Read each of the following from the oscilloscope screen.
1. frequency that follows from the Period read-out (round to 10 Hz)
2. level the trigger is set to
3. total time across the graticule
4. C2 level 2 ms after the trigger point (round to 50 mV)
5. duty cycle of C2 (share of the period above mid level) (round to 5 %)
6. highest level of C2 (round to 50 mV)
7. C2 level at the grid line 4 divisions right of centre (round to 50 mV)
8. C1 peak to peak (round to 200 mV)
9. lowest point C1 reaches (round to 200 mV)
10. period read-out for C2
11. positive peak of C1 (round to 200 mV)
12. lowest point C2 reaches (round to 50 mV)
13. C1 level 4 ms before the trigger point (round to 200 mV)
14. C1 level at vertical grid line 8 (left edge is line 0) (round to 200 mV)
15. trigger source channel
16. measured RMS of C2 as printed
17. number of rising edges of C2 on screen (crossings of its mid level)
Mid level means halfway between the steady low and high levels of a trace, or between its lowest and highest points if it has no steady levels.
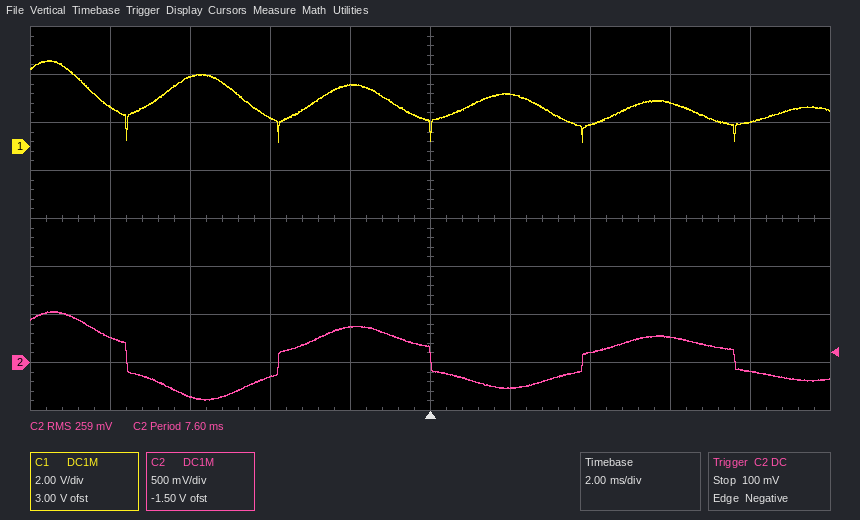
130 Hz
100 mV
20 ms
-250 mV
50 %
550 mV
-100 mV
3.4 V
200 mV
7.60 ms
3.6 V
-400 mV
1.2 V
1.8 V
C2
259 mV
2
